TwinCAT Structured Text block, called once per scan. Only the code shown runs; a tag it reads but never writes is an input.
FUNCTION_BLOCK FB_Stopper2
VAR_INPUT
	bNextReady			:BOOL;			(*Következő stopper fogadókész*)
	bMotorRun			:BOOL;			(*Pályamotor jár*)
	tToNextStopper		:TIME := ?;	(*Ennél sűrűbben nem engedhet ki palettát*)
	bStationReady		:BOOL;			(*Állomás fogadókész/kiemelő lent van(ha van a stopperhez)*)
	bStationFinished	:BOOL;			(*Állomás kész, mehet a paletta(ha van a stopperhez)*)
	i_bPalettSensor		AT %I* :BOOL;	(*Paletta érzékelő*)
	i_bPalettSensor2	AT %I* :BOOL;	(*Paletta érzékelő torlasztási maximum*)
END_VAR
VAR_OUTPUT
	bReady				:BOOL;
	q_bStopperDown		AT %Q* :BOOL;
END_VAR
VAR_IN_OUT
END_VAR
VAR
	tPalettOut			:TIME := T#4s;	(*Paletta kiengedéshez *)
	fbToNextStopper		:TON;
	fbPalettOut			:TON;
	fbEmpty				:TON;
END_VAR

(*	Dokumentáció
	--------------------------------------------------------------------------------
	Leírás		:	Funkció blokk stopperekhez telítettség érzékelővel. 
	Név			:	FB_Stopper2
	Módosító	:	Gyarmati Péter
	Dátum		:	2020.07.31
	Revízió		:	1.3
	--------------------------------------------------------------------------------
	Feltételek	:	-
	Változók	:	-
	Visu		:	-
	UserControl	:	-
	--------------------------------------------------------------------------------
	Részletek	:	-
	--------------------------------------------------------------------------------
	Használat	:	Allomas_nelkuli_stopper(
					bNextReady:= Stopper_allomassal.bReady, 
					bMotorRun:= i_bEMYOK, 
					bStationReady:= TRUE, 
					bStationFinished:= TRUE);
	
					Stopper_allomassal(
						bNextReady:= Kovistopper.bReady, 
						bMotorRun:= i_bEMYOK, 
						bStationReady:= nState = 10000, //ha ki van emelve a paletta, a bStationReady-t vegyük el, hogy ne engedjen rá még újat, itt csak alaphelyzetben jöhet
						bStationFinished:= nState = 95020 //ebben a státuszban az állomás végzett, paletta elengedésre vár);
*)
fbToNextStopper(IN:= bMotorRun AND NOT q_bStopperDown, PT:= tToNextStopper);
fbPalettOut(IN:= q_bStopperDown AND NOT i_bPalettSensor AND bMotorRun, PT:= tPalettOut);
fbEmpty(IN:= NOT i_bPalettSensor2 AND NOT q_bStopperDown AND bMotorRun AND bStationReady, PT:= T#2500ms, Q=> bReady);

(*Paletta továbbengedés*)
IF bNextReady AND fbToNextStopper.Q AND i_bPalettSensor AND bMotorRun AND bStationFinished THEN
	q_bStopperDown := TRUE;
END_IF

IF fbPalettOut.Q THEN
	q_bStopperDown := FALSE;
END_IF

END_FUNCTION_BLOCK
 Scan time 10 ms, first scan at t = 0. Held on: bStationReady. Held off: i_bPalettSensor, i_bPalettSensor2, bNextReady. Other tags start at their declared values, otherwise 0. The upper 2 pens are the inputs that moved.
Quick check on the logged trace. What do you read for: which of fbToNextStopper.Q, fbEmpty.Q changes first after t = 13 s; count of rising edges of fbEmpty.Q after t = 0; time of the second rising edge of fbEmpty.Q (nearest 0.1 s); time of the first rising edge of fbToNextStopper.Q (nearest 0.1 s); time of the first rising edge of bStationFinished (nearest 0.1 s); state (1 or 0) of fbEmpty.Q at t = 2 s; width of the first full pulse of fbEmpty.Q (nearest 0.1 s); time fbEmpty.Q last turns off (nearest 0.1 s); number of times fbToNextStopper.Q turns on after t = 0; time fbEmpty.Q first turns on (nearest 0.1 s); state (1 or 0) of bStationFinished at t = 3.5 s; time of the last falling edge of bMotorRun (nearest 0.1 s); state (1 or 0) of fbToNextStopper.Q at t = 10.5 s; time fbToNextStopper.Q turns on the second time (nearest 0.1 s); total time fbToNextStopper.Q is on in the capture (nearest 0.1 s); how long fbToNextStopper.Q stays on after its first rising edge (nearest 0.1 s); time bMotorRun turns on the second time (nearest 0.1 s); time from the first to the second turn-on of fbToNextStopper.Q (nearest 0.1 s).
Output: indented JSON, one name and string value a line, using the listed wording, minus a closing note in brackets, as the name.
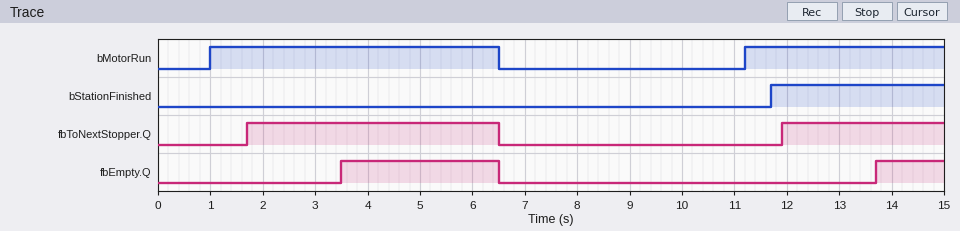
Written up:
{
  "which of fbToNextStopper.Q, fbEmpty.Q changes first after t = 13 s": "fbEmpty.Q",
  "count of rising edges of fbEmpty.Q after t = 0": "2",
  "time of the second rising edge of fbEmpty.Q": "13.7 s",
  "time of the first rising edge of fbToNextStopper.Q": "1.7 s",
  "time of the first rising edge of bStationFinished": "11.7 s",
  "state (1 or 0) of fbEmpty.Q at t = 2 s": "0",
  "width of the first full pulse of fbEmpty.Q": "3.0 s",
  "time fbEmpty.Q last turns off": "6.5 s",
  "number of times fbToNextStopper.Q turns on after t = 0": "2",
  "time fbEmpty.Q first turns on": "3.5 s",
  "state (1 or 0) of bStationFinished at t = 3.5 s": "0",
  "time of the last falling edge of bMotorRun": "6.5 s",
  "state (1 or 0) of fbToNextStopper.Q at t = 10.5 s": "0",
  "time fbToNextStopper.Q turns on the second time": "11.9 s",
  "total time fbToNextStopper.Q is on in the capture": "7.9 s",
  "how long fbToNextStopper.Q stays on after its first rising edge": "4.8 s",
  "time bMotorRun turns on the second time": "11.2 s",
  "time from the first to the second turn-on of fbToNextStopper.Q": "10.2 s"
}
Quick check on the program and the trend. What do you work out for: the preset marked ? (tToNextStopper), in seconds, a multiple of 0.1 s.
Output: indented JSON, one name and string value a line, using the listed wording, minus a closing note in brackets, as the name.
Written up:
{
  "the preset marked ? (tToNextStopper), in seconds, a multiple of 0.1 s": "0.7 s"
}
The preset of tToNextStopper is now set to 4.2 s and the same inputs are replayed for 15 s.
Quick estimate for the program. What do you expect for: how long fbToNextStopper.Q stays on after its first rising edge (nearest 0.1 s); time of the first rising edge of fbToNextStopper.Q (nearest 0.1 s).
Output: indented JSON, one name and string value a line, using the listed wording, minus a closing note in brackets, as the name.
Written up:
{
  "how long fbToNextStopper.Q stays on after its first rising edge": "1.3 s",
  "time of the first rising edge of fbToNextStopper.Q": "5.2 s"
}
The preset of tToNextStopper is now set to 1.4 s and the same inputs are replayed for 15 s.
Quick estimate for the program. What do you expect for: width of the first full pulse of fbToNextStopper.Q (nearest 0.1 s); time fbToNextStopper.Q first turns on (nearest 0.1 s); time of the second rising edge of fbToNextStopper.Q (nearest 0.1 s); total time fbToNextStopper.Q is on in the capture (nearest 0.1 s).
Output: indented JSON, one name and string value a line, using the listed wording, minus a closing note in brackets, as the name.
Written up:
{
  "width of the first full pulse of fbToNextStopper.Q": "4.1 s",
  "time fbToNextStopper.Q first turns on": "2.4 s",
  "time of the second rising edge of fbToNextStopper.Q": "12.6 s",
  "total time fbToNextStopper.Q is on in the capture": "6.5 s"
}
